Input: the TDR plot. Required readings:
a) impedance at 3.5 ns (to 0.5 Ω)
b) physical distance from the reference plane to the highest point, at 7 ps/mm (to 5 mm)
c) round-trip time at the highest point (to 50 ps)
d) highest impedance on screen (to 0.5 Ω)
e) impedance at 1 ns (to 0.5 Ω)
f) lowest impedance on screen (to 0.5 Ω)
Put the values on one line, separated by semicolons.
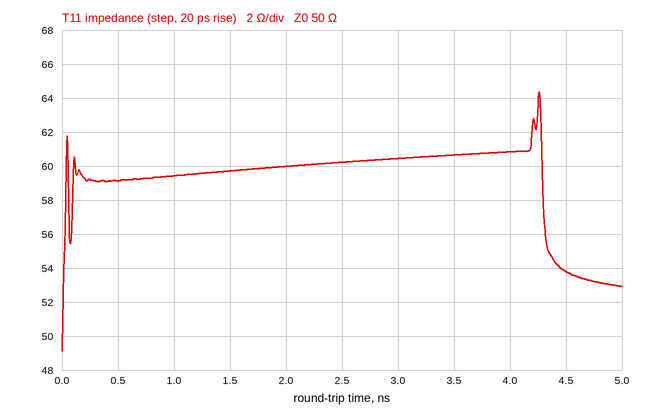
60.5 Ω; 305 mm; 4.25 ns; 64.5 Ω; 59.5 Ω; 49.0 Ω
